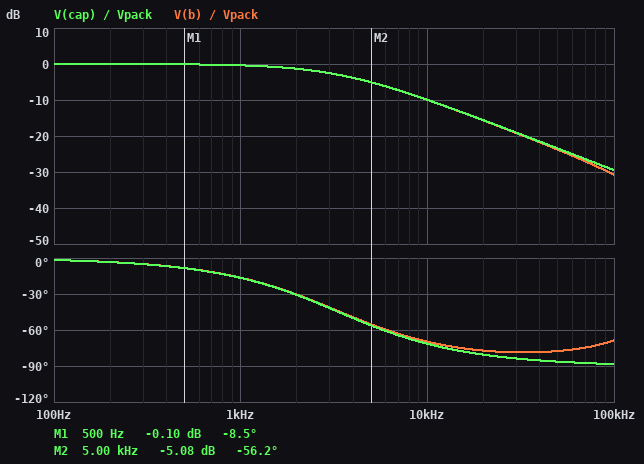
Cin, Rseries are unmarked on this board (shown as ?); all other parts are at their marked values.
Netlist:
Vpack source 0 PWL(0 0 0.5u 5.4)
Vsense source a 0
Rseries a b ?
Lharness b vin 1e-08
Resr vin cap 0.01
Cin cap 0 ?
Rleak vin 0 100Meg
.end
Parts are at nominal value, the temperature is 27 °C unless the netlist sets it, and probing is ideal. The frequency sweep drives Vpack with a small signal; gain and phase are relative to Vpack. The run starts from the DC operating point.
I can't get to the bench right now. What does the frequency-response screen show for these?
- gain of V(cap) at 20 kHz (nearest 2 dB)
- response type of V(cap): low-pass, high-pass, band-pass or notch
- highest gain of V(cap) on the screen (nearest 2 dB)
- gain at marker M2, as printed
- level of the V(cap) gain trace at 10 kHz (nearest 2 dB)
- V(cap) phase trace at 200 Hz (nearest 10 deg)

-16 dB
low-pass
0 dB
-5.08 dB
-10 dB
0 deg
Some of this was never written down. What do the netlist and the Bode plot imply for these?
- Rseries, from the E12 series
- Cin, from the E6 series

1 Ω
47 µF
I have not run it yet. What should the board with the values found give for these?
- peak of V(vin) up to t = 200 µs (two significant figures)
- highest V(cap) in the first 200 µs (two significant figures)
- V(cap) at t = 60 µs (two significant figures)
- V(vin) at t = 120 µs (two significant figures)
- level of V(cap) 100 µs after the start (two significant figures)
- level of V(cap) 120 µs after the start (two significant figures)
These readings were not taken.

5.3 V
5.3 V
3.9 V
5.0 V
4.7 V
5.0 V
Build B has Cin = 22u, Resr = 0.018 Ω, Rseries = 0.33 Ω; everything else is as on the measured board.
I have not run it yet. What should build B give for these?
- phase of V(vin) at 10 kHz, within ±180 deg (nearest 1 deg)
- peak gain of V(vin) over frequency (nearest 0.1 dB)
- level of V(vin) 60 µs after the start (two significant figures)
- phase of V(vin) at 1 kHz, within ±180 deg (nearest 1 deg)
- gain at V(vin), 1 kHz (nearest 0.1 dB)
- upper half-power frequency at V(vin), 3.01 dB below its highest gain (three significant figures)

-24 deg
0 dB
5.4 V
-3 deg
0 dB
20.9 kHz
